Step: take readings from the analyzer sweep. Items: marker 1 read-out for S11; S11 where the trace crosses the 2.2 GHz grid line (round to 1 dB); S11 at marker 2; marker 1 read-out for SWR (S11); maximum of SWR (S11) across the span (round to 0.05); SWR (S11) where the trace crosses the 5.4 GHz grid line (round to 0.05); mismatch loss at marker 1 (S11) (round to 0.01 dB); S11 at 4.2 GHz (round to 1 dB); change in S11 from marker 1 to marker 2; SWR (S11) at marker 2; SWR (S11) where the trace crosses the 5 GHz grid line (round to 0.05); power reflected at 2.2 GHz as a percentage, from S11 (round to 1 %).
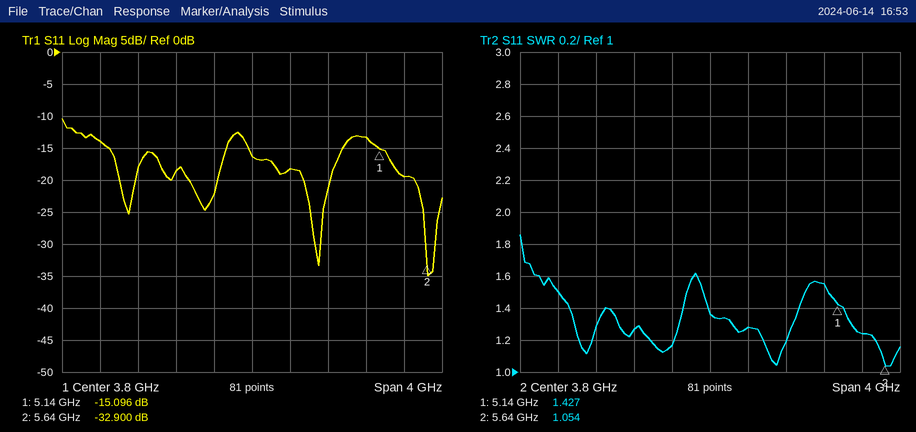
-15.096 dB
-14 dB
-32.900 dB
1.427
1.85
1.25
0.14 dB
-18 dB
-17.804 dB
1.054
1.55
4 %
